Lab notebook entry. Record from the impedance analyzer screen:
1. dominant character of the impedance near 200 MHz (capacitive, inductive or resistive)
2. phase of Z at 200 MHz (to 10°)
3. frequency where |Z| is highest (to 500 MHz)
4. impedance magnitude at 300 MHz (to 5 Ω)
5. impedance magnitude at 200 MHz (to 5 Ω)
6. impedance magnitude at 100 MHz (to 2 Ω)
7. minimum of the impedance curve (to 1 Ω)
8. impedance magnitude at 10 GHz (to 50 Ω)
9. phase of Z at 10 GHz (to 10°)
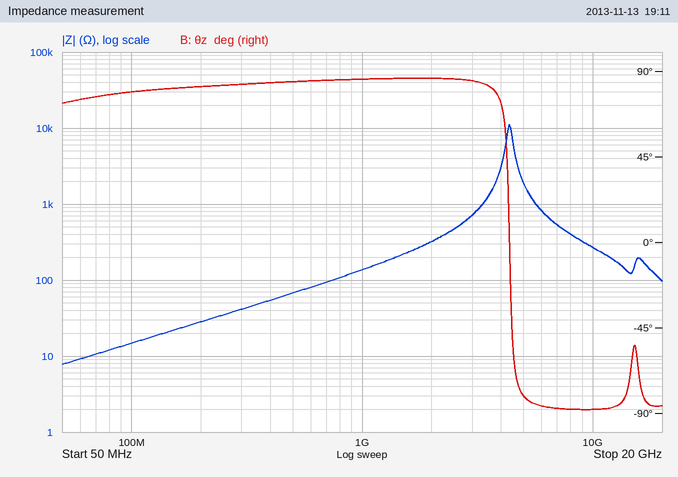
inductive
80°
4.5 GHz
40 Ω
30 Ω
14 Ω
8 Ω
250 Ω
-90°
